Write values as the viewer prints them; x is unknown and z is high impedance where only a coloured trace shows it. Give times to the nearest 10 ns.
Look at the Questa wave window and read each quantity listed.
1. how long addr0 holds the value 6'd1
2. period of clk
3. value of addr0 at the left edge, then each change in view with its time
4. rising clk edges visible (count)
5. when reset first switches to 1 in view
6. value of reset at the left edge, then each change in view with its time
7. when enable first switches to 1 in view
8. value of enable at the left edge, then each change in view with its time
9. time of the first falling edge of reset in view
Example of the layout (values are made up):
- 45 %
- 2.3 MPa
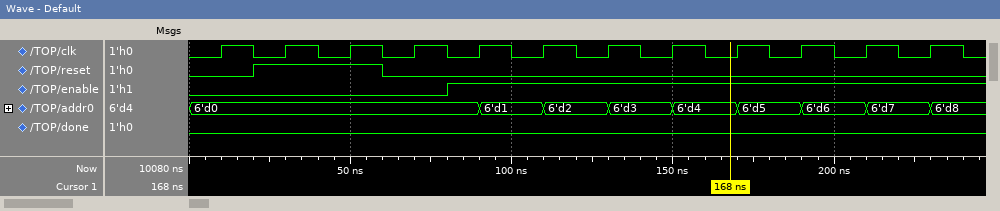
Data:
- 20 ns
- 20 ns
- 6'd0, 6'd1 at 90 ns, 6'd2 at 110 ns, 6'd3 at 130 ns, 6'd4 at 150 ns, 6'd5 at 170 ns, 6'd6 at 190 ns, 6'd7 at 210 ns, 6'd8 at 230 ns
- 12
- 20 ns
- 0, 1 at 20 ns, 0 at 60 ns
- 80 ns
- 0, 1 at 80 ns
- 60 ns
